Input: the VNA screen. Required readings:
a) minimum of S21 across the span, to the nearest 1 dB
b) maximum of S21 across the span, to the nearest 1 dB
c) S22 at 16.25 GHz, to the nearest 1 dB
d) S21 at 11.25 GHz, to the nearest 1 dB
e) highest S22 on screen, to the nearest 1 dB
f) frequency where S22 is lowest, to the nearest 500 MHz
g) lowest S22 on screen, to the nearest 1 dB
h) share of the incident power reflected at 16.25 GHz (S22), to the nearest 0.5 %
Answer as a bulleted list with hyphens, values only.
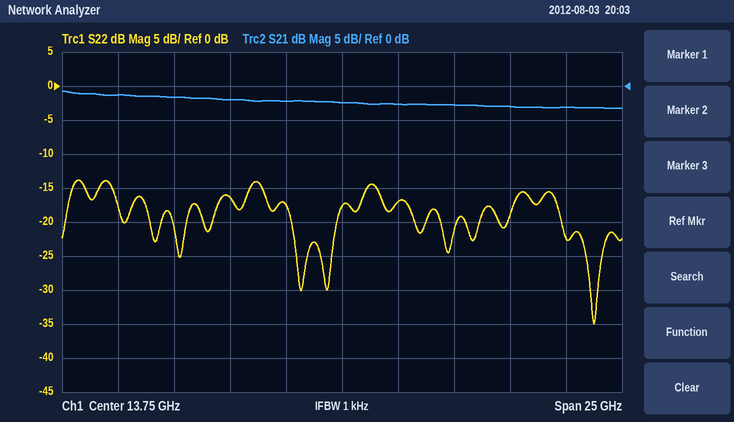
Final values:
- -3 dB
- -1 dB
- -17 dB
- -2 dB
- -14 dB
- 25.0 GHz
- -35 dB
- 2.0 %
